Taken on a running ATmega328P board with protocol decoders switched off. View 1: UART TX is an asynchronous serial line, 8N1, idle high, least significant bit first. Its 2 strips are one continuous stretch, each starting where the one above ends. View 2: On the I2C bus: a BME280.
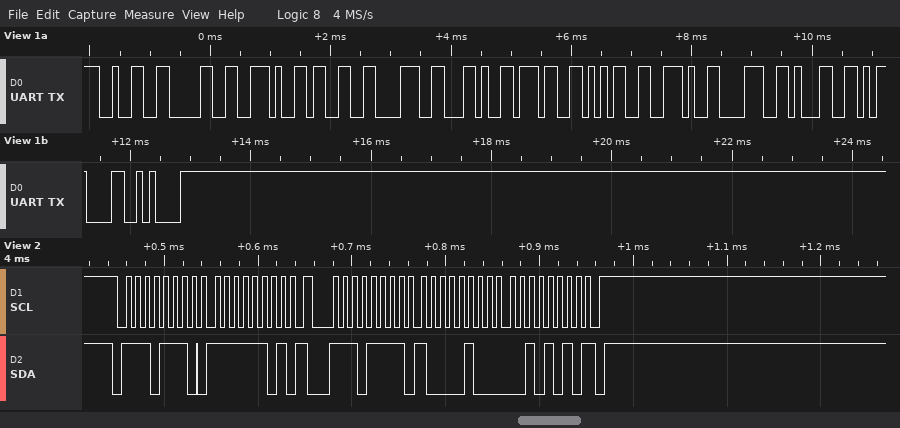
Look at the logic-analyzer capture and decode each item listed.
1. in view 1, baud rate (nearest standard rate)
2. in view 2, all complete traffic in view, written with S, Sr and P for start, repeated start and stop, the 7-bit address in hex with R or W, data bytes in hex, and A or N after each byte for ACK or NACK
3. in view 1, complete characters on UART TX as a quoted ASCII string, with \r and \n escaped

9600 baud
S 77W A FD A Sr 77R A 84 A 2A N P
"20.38,75.81\r\n"
